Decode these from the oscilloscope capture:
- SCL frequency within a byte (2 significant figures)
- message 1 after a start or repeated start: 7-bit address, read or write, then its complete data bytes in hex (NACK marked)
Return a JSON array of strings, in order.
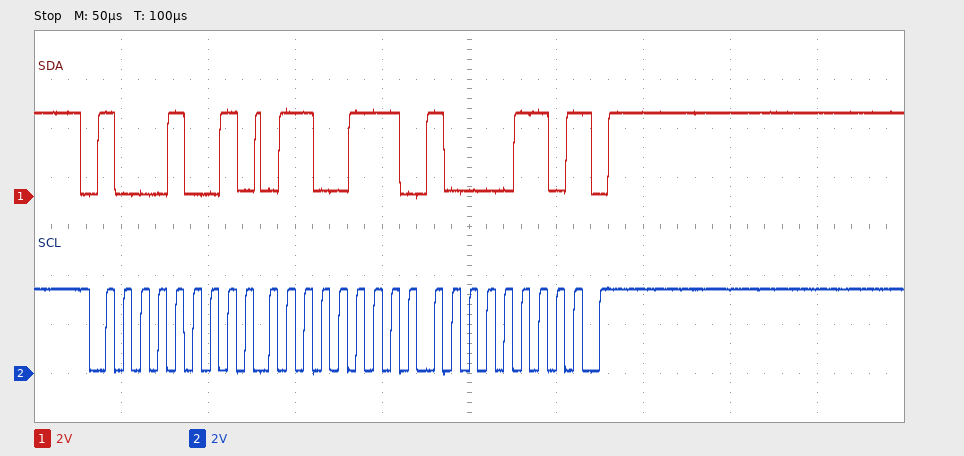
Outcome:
["100 kHz", "0x44 read: 67 86 NACK"]
